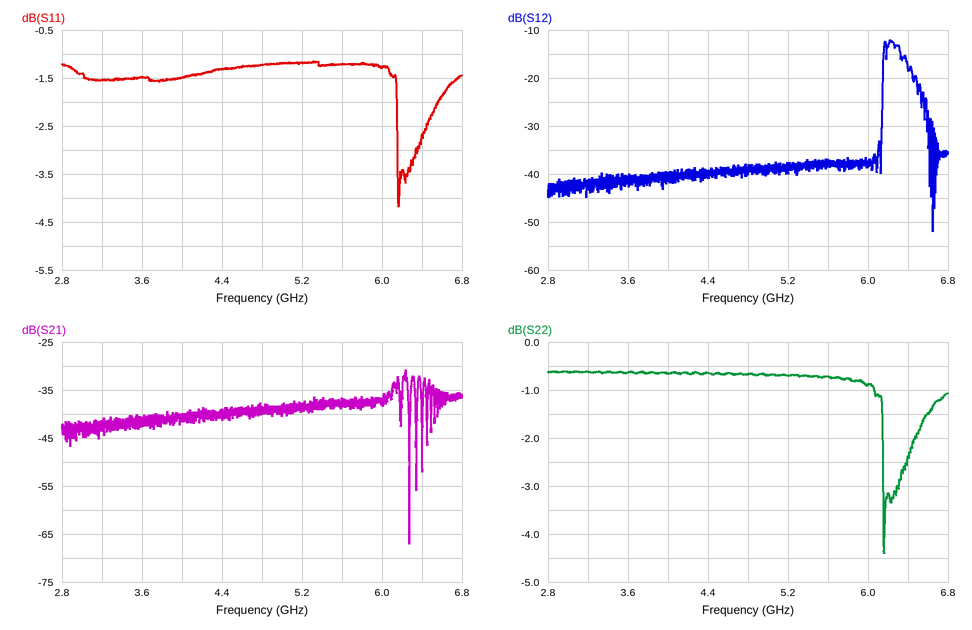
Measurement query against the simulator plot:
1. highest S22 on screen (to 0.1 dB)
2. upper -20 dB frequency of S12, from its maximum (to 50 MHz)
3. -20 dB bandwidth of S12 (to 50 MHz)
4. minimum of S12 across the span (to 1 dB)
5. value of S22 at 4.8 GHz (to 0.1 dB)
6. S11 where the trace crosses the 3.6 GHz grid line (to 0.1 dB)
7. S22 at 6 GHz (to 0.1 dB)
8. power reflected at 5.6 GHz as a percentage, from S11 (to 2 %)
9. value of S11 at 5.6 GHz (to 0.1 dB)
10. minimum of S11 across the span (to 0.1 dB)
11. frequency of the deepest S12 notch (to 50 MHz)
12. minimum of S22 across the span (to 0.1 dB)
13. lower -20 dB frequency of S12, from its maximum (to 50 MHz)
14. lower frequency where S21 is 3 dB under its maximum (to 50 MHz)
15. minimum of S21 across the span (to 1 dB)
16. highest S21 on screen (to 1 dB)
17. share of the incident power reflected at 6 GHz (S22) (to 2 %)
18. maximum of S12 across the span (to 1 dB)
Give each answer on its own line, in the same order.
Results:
-0.6 dB
6.60 GHz
450 MHz
-52 dB
-0.7 dB
-1.5 dB
-0.9 dB
76 %
-1.2 dB
-4.2 dB
6.65 GHz
-4.4 dB
6.15 GHz
6.20 GHz
-67 dB
-31 dB
82 %
-12 dB
